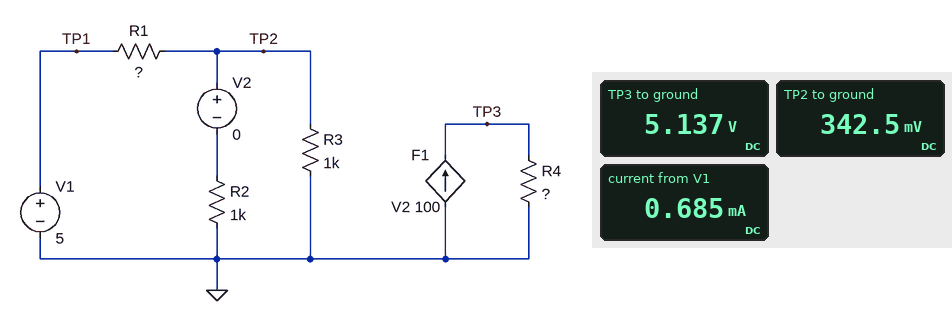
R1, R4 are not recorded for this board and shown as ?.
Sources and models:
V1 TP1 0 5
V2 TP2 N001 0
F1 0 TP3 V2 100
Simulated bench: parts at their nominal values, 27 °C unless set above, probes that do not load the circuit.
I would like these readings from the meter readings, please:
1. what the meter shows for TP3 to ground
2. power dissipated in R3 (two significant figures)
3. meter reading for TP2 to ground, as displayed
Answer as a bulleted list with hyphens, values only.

- 5.137 V
- 120 µW
- 342.5 mV
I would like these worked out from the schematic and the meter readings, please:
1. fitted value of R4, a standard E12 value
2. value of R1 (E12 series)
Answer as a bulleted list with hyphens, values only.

- 150 Ω
- 6.8 kΩ
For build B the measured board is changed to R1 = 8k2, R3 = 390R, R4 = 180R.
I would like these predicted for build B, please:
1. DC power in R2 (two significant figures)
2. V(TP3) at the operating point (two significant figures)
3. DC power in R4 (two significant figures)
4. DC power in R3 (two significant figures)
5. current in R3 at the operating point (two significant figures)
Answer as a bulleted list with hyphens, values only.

- 27 µW
- 3.0 V
- 49 mW
- 70 µW
- 420 µA
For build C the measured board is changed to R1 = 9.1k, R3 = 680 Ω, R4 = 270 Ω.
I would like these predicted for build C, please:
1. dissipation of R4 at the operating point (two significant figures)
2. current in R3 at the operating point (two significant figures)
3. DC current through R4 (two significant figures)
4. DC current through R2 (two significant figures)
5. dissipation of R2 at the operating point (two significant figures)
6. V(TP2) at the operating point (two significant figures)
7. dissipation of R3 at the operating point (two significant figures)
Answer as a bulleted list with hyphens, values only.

- 120 mW
- 310 µA
- 21 mA
- 210 µA
- 45 µW
- 210 mV
- 67 µW
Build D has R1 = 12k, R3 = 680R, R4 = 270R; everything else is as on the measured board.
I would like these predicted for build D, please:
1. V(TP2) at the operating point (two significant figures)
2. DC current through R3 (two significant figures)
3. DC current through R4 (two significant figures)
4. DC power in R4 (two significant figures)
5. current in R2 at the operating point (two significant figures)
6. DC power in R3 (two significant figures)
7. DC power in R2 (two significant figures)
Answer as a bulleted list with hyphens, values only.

- 160 mV
- 240 µA
- 16 mA
- 72 mW
- 160 µA
- 39 µW
- 27 µW
